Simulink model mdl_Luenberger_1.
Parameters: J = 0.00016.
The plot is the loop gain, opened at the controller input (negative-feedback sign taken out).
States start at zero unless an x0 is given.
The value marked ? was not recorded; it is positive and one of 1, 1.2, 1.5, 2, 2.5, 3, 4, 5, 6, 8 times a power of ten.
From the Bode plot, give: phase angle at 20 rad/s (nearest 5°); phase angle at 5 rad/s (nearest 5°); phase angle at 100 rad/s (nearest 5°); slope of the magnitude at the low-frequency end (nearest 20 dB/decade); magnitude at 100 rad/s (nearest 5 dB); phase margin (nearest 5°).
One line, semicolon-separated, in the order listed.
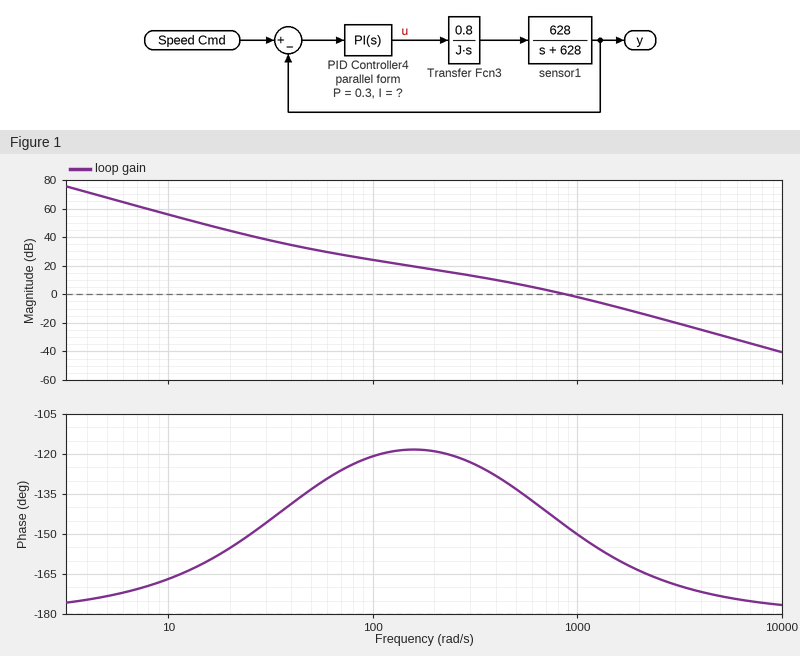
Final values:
-155°; -175°; -120°; -40 dB/decade; 25 dB; 35°
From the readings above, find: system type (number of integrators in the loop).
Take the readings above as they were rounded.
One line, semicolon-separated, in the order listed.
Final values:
2
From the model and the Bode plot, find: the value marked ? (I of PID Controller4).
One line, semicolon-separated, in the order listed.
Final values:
12
